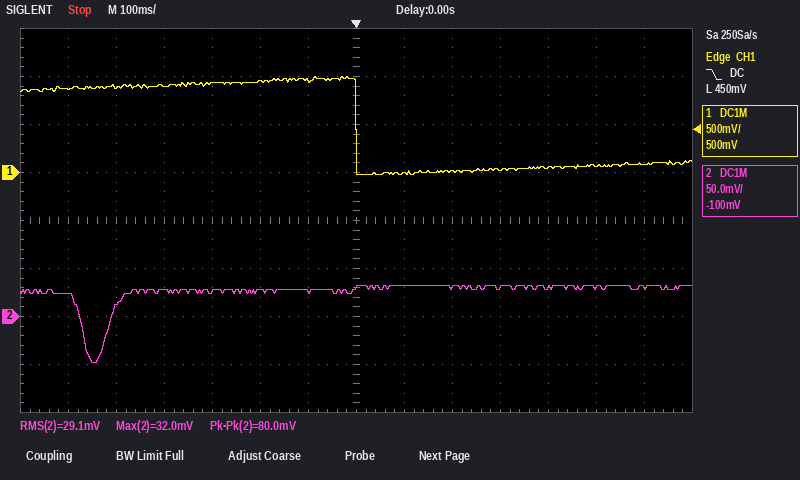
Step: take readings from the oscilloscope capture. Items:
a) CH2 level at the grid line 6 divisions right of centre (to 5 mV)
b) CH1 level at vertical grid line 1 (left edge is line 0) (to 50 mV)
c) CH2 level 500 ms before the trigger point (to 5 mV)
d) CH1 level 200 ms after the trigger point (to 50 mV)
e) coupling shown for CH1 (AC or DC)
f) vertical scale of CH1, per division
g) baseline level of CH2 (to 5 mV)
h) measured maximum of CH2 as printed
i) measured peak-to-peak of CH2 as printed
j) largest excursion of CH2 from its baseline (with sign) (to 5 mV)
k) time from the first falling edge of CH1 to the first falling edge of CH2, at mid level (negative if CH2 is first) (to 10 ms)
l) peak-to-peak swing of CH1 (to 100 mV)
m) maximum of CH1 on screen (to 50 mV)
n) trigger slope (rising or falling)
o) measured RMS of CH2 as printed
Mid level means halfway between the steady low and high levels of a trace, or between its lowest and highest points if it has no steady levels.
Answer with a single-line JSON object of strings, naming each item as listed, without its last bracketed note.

{"CH2 level at the grid line 6 divisions right of centre": "30 mV", "CH1 level at vertical grid line 1 (left edge is line 0)": "850 mV", "CH2 level 500 ms before the trigger point": "10 mV", "CH1 level 200 ms after the trigger point": "0 mV", "coupling shown for CH1": "DC", "vertical scale of CH1, per division": "500 mV", "baseline level of CH2": "30 mV", "measured maximum of CH2 as printed": "32.0 mV", "measured peak-to-peak of CH2 as printed": "80.0 mV", "largest excursion of CH2 from its baseline (with sign)": "-75 mV", "time from the first falling edge of CH1 to the first falling edge of CH2, at mid level (negative if CH2 is first)": "-570 ms", "peak-to-peak swing of CH1": "1.00 V", "maximum of CH1 on screen": "1.00 V", "trigger slope": "falling", "measured RMS of CH2 as printed": "29.1 mV"}
